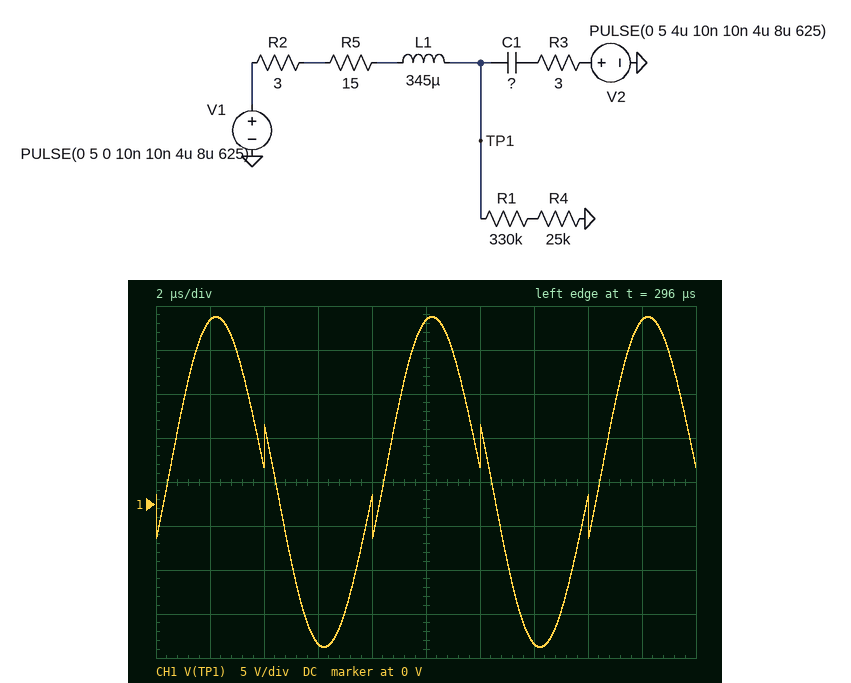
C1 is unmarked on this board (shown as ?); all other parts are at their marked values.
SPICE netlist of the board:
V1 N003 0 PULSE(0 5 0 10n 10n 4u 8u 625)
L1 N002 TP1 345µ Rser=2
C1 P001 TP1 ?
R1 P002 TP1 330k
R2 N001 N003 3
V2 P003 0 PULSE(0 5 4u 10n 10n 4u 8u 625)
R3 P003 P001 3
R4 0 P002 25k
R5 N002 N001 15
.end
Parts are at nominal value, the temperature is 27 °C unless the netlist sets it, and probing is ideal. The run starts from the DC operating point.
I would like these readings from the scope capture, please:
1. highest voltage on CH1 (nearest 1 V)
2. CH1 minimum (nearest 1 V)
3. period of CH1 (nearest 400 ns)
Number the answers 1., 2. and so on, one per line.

1. 21 V
2. -16 V
3. 8.0 µs
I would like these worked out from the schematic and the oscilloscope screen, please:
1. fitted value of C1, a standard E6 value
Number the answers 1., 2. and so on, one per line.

1. 3.3 nF
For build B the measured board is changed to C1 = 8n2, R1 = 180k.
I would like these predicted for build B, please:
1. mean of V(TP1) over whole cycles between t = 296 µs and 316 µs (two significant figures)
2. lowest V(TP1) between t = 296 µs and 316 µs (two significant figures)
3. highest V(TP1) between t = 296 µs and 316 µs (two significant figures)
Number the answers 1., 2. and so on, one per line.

1. 2.5 V
2. -8.3 V
3. 13 V
